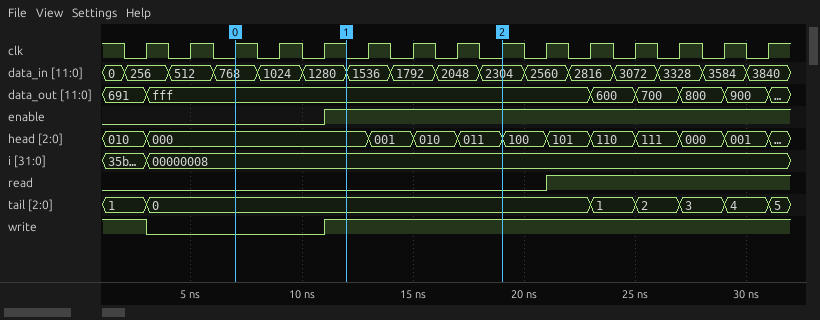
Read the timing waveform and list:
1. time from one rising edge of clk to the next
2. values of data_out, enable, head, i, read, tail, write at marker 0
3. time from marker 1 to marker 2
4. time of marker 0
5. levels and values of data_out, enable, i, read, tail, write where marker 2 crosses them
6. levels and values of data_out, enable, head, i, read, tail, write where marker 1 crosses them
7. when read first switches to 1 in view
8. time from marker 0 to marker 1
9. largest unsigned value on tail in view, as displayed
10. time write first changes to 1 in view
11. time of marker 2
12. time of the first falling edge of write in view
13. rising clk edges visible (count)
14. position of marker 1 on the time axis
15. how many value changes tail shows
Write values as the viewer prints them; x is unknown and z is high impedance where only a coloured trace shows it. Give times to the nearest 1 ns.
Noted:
2 ns
data_out=fff, enable=0, head=000, i=00000008, read=0, tail=0, write=0
7 ns
7 ns
data_out=fff, enable=1, i=00000008, read=0, tail=0, write=1
data_out=fff, enable=1, head=000, i=00000008, read=0, tail=0, write=1
21 ns
5 ns
5
11 ns
19 ns
3 ns
15
12 ns
6
